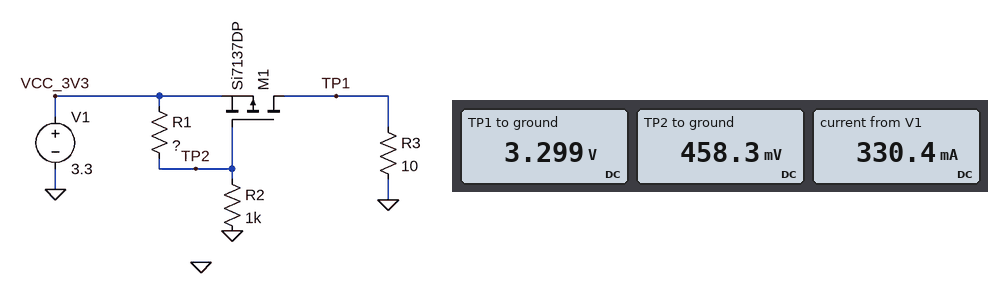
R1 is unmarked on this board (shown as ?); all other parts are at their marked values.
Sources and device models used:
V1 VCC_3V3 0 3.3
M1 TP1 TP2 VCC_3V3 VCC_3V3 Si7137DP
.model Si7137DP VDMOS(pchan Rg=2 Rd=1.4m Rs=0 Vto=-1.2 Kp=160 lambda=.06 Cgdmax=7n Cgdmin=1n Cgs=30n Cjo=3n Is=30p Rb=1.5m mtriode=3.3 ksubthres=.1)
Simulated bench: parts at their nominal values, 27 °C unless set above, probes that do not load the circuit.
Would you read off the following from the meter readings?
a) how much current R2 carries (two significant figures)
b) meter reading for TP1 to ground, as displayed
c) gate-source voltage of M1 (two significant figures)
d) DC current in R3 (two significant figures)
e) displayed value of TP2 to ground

460 µA
3.299 V
-2.8 V
330 mA
458.3 mV
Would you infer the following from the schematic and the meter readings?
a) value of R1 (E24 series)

6.2 kΩ
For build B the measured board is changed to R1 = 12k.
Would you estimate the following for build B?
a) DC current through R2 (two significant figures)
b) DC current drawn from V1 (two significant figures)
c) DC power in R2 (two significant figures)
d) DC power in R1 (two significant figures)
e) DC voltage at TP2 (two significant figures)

250 µA
330 mA
64 µW
770 µW
250 mV
